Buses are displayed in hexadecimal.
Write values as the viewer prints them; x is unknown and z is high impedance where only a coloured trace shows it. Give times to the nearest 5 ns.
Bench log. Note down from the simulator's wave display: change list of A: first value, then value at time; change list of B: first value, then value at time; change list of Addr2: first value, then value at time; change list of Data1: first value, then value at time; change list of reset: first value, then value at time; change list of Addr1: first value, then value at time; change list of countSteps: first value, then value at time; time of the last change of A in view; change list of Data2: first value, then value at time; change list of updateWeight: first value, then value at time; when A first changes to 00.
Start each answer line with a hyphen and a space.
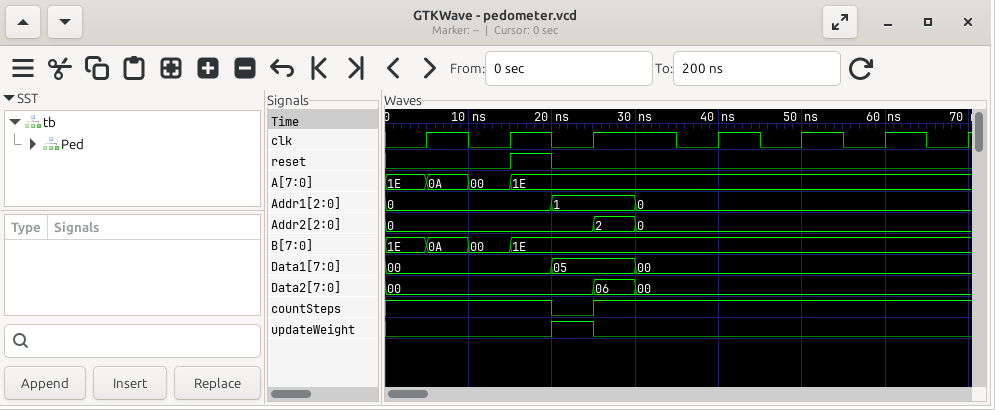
- 1E, 0A at 5 ns, 00 at 10 ns, 1E at 15 ns
- 1E, 0A at 5 ns, 00 at 10 ns, 1E at 15 ns
- 0, 2 at 25 ns, 0 at 30 ns
- 00, 05 at 20 ns, 00 at 30 ns
- 0, 1 at 15 ns, 0 at 20 ns
- 0, 1 at 20 ns, 0 at 30 ns
- 1, 0 at 20 ns, 1 at 25 ns
- 15 ns
- 00, 06 at 25 ns, 00 at 30 ns
- 0, 1 at 20 ns, 0 at 25 ns
- 10 ns
